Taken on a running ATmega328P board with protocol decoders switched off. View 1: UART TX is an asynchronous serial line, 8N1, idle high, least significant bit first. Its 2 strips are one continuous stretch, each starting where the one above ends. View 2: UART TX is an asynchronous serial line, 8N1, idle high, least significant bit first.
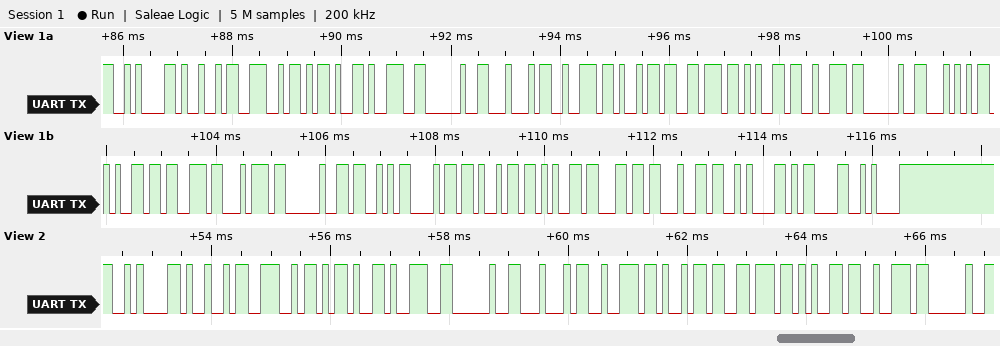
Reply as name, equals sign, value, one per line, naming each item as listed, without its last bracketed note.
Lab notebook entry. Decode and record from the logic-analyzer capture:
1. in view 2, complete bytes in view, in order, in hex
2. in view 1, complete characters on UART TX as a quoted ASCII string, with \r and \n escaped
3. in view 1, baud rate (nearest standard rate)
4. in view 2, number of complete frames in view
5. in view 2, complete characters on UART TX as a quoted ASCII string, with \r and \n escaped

in view 2, complete bytes in view, in order, in hex = 0A 49 4E 2D 39 20 44 72 69 76 65 72 20
in view 1, complete characters on UART TX as a quoted ASCII string, with \r and \n escaped = "\nIN-9 Driver Test Shield\n\r\n"
in view 1, baud rate = 9600 baud
in view 2, number of complete frames in view = 13
in view 2, complete characters on UART TX as a quoted ASCII string, with \r and \n escaped = "\nIN-9 Driver "
